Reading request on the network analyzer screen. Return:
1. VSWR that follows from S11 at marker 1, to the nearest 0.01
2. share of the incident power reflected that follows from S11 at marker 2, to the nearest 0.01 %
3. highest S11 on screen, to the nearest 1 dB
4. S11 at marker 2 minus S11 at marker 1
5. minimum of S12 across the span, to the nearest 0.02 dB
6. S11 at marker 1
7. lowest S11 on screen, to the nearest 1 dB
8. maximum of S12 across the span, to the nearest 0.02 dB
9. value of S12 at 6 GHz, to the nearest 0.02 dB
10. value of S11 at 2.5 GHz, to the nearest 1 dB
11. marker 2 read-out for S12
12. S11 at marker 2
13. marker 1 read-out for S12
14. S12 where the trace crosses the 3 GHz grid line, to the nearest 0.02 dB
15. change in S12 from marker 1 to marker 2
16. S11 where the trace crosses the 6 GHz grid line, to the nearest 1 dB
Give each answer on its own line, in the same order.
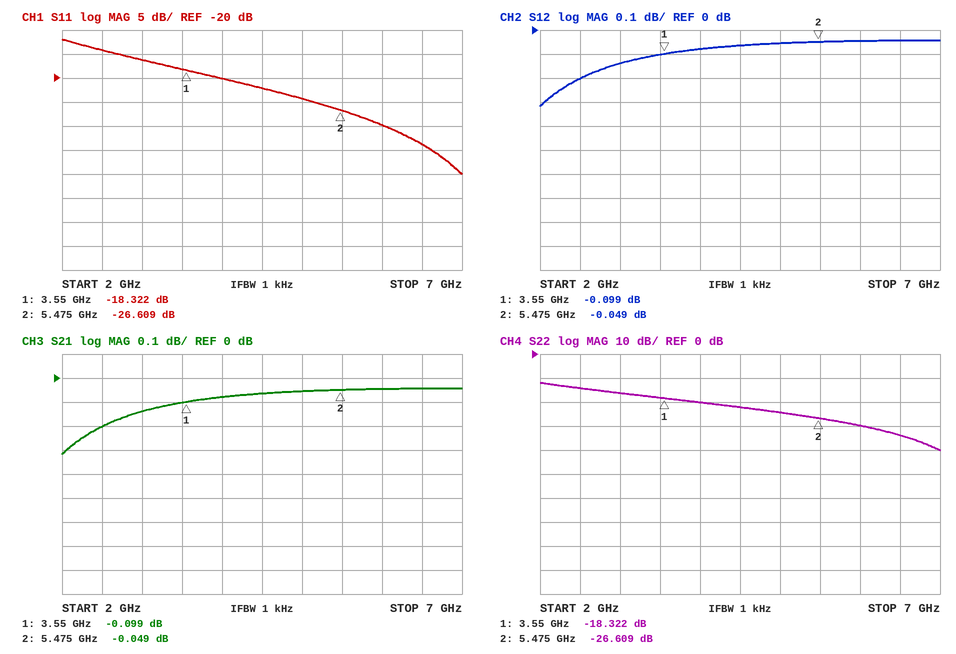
1.28
0.22 %
-12 dB
-8.287 dB
-0.32 dB
-18.322 dB
-40 dB
-0.04 dB
-0.04 dB
-14 dB
-0.049 dB
-26.609 dB
-0.099 dB
-0.14 dB
0.050 dB
-30 dB
